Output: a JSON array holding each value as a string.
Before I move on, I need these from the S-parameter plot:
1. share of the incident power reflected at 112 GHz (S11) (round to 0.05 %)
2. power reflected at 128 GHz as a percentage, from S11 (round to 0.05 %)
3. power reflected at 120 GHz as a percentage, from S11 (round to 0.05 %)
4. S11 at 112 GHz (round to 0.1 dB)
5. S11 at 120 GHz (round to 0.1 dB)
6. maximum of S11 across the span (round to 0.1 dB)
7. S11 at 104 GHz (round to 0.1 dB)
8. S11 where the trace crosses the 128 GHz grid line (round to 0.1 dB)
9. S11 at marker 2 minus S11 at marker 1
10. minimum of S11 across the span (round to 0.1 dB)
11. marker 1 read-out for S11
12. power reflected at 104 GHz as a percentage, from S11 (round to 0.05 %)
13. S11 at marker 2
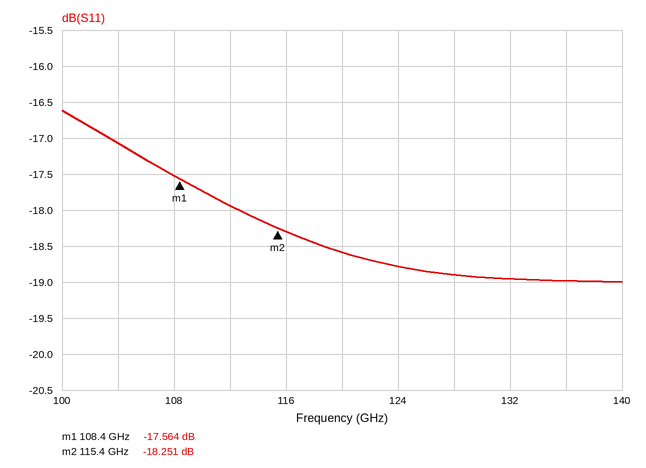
["1.60 %", "1.30 %", "1.40 %", "-17.9 dB", "-18.6 dB", "-16.6 dB", "-17.1 dB", "-18.9 dB", "-0.687 dB", "-19.0 dB", "-17.564 dB", "1.95 %", "-18.251 dB"]
